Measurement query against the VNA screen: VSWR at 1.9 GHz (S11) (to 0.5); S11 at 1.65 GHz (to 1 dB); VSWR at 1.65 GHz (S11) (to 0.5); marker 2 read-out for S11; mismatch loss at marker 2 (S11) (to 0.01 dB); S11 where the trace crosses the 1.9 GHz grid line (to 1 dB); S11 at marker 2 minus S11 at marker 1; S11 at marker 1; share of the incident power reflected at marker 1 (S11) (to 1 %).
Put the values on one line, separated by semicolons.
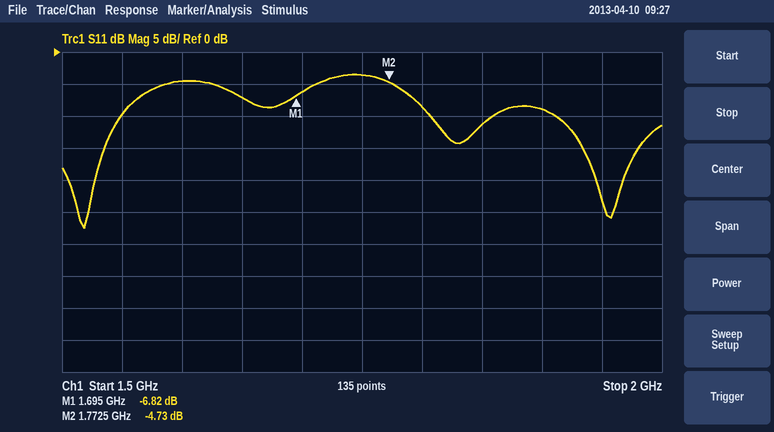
2.0; -7 dB; 2.5; -4.73 dB; 1.78 dB; -9 dB; 2.09 dB; -6.82 dB; 21 %
